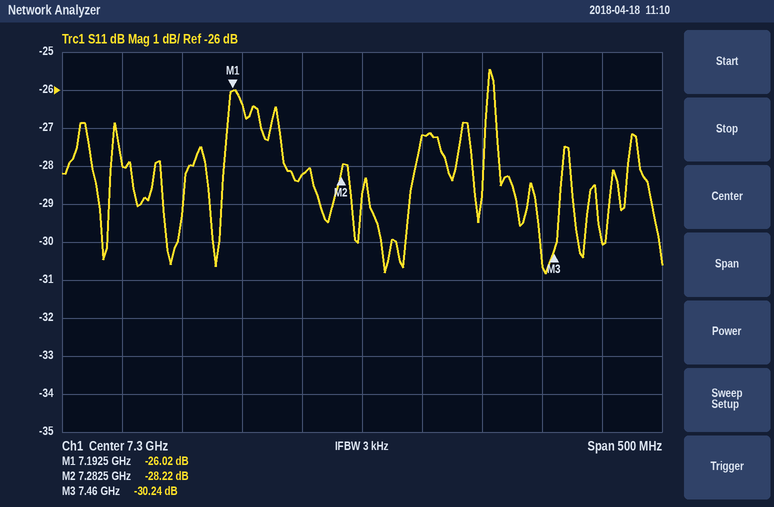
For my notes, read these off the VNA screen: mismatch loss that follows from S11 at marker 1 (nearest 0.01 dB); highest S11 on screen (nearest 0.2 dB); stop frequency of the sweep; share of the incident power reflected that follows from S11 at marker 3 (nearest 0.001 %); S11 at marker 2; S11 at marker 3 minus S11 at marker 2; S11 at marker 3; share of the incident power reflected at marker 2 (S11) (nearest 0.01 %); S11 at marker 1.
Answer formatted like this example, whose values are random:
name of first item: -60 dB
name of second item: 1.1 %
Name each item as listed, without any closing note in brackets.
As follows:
mismatch loss that follows from S11 at marker 1: 0.01 dB
highest S11 on screen: -25.4 dB
stop frequency of the sweep: 7.55 GHz
share of the incident power reflected that follows from S11 at marker 3: 0.095 %
S11 at marker 2: -28.22 dB
S11 at marker 3 minus S11 at marker 2: -2.02 dB
S11 at marker 3: -30.24 dB
share of the incident power reflected at marker 2 (S11): 0.15 %
S11 at marker 1: -26.02 dB
